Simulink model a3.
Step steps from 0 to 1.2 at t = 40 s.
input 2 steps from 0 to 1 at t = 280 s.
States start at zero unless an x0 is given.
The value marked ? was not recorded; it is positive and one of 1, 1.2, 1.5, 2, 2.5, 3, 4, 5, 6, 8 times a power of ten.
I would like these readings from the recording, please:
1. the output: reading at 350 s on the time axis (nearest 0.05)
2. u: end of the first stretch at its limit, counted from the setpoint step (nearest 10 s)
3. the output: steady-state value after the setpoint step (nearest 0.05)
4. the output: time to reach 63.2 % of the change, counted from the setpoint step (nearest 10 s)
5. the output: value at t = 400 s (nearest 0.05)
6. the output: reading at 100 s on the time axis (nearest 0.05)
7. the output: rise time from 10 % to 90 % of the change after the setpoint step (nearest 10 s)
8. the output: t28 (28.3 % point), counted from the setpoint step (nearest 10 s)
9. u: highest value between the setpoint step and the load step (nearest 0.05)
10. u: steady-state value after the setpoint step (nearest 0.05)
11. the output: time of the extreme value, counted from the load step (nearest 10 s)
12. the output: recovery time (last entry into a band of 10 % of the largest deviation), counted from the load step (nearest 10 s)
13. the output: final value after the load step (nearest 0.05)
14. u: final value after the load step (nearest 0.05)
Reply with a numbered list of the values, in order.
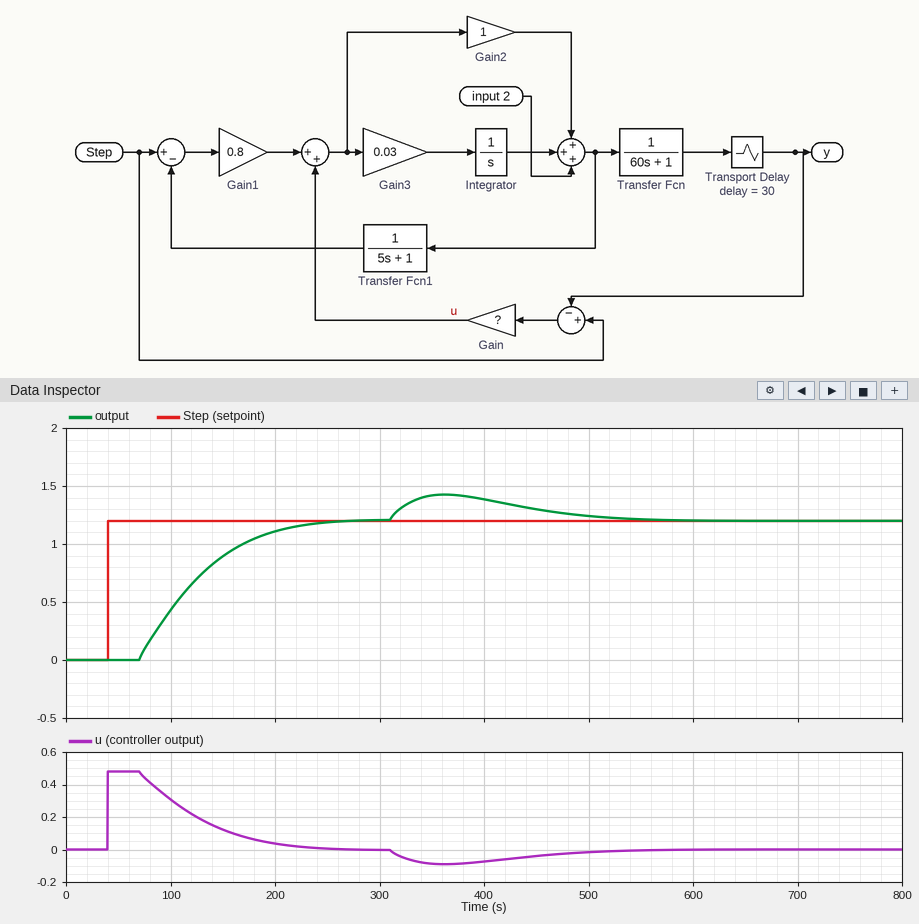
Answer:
1. 1.40
2. 30 s
3. 1.20
4. 90 s
5. 1.40
6. 0.45
7. 110 s
8. 50 s
9. 0.50
10. 0.00
11. 80 s
12. 250 s
13. 1.20
14. 0.00
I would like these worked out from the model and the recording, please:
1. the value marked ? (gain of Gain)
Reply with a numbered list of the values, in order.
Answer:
1. 0.4
